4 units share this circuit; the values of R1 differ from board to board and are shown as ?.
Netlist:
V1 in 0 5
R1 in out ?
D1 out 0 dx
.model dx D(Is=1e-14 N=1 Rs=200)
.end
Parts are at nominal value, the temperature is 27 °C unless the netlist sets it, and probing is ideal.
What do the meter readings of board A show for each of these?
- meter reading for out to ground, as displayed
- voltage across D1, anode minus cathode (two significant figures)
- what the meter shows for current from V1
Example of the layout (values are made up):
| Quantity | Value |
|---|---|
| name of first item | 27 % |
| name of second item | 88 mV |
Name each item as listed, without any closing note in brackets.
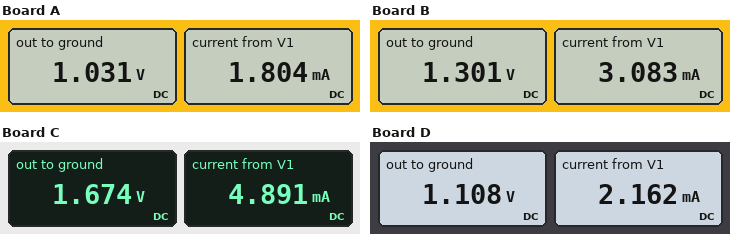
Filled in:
| Quantity | Value |
|---|---|
| meter reading for out to ground, as displayed | 1.031 V |
| voltage across D1, anode minus cathode | 1.0 V |
| what the meter shows for current from V1 | 1.804 mA |
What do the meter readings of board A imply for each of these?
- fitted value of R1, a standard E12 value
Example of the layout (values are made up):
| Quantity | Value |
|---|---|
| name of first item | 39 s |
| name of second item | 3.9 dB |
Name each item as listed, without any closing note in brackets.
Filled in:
| Quantity | Value |
|---|---|
| fitted value of R1, a standard E12 value | 2.2 kΩ |
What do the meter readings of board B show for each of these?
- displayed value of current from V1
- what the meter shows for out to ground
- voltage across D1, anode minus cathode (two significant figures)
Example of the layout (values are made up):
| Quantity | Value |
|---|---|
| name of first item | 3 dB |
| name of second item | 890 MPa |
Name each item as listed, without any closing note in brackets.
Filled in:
| Quantity | Value |
|---|---|
| displayed value of current from V1 | 3.083 mA |
| what the meter shows for out to ground | 1.301 V |
| voltage across D1, anode minus cathode | 1.3 V |
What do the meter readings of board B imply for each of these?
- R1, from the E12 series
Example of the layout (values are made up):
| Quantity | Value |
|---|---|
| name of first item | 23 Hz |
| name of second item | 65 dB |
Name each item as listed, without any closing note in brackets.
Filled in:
| Quantity | Value |
|---|---|
| R1, from the E12 series | 1.2 kΩ |
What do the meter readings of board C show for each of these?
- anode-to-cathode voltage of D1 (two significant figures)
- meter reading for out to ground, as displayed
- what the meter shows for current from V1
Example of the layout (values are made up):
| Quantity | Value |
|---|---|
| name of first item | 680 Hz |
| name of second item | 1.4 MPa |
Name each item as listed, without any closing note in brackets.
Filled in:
| Quantity | Value |
|---|---|
| anode-to-cathode voltage of D1 | 1.7 V |
| meter reading for out to ground, as displayed | 1.674 V |
| what the meter shows for current from V1 | 4.891 mA |
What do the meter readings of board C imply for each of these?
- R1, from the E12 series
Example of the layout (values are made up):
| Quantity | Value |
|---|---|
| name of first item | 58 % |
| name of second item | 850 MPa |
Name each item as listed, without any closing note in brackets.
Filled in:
| Quantity | Value |
|---|---|
| R1, from the E12 series | 680 Ω |
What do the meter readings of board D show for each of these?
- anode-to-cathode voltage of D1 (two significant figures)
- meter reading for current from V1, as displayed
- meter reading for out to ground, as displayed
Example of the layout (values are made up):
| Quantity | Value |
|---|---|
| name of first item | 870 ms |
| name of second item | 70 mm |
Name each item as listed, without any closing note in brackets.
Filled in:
| Quantity | Value |
|---|---|
| anode-to-cathode voltage of D1 | 1.1 V |
| meter reading for current from V1, as displayed | 2.162 mA |
| meter reading for out to ground, as displayed | 1.108 V |
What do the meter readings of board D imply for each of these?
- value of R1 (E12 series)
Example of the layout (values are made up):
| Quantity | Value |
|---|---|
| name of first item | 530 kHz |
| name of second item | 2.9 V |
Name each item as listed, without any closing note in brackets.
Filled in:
| Quantity | Value |
|---|---|
| value of R1 | 1.8 kΩ |
